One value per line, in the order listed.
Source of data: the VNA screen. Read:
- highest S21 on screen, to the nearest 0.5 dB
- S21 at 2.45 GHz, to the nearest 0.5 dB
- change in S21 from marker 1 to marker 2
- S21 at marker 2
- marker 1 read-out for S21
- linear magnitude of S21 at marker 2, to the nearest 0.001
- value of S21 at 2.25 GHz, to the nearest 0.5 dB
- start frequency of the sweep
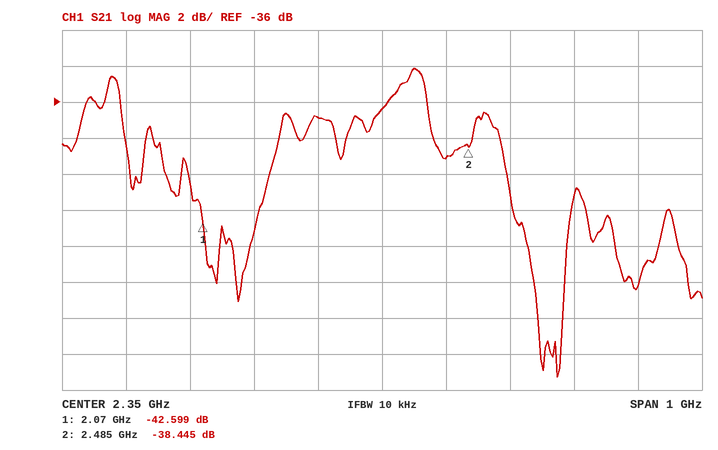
-34.0 dB
-39.0 dB
4.154 dB
-38.445 dB
-42.599 dB
0.012
-37.0 dB
1.85 GHz
